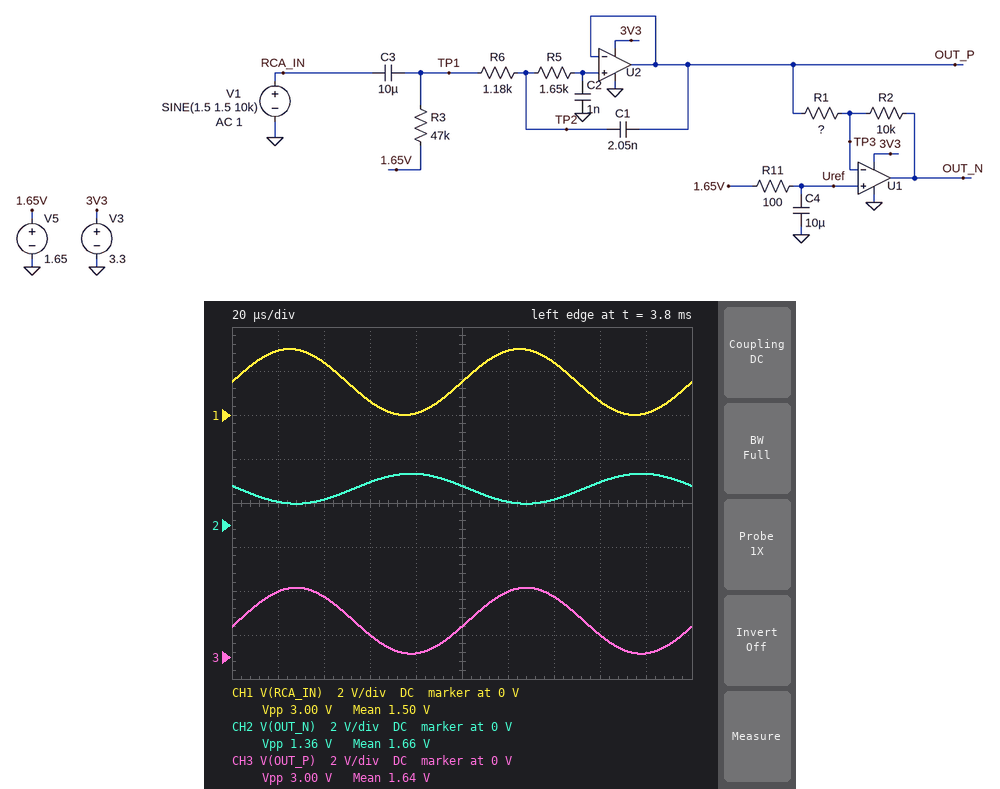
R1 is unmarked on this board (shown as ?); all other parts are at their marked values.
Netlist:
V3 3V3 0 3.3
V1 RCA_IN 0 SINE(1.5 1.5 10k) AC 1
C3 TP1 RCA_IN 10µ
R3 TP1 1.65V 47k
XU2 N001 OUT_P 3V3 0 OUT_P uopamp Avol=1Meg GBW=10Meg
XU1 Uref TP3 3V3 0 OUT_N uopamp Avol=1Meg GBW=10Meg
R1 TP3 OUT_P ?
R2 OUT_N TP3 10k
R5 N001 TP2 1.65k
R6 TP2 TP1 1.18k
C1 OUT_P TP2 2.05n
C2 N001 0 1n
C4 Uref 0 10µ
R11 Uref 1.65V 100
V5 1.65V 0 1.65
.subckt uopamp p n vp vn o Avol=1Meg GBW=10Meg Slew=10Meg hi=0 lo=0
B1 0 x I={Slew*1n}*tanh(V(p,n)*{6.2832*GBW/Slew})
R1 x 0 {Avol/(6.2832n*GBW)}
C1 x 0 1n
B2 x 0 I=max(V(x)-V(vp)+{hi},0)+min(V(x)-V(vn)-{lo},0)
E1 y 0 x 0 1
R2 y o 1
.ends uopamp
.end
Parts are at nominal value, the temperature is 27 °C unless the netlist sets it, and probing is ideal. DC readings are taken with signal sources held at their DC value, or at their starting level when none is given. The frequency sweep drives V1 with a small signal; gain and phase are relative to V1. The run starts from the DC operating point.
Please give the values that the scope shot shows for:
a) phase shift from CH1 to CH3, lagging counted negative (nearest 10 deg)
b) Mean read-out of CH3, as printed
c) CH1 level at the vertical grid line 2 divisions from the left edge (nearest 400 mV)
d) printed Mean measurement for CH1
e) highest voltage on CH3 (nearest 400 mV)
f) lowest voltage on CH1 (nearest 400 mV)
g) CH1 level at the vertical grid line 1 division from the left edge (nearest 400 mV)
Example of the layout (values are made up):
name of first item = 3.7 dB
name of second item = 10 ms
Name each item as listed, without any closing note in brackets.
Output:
phase shift from CH1 to CH3, lagging counted negative = -10 deg
Mean read-out of CH3, as printed = 1.64 V
CH1 level at the vertical grid line 2 divisions from the left edge = 2.4 V
printed Mean measurement for CH1 = 1.50 V
highest voltage on CH3 = 3.2 V
lowest voltage on CH1 = 0 V
CH1 level at the vertical grid line 1 division from the left edge = 2.8 V
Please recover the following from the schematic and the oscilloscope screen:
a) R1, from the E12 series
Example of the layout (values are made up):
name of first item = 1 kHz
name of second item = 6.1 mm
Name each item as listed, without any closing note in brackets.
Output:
R1, from the E12 series = 22 kΩ
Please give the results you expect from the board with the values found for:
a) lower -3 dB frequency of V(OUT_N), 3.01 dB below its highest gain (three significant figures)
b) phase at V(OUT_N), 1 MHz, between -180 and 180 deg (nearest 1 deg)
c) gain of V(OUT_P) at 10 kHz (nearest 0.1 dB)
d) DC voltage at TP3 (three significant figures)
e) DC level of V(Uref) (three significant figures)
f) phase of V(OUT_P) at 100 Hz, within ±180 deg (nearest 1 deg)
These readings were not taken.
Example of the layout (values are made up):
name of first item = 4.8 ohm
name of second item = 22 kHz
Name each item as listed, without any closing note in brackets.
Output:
lower -3 dB frequency of V(OUT_N), 3.01 dB below its highest gain = 339 mHz
phase at V(OUT_N), 1 MHz, between -180 and 180 deg = -8 deg
gain of V(OUT_P) at 10 kHz = 0 dB
DC voltage at TP3 = 1.65 V
DC level of V(Uref) = 1.65 V
phase of V(OUT_P) at 100 Hz, within ±180 deg = 0 deg
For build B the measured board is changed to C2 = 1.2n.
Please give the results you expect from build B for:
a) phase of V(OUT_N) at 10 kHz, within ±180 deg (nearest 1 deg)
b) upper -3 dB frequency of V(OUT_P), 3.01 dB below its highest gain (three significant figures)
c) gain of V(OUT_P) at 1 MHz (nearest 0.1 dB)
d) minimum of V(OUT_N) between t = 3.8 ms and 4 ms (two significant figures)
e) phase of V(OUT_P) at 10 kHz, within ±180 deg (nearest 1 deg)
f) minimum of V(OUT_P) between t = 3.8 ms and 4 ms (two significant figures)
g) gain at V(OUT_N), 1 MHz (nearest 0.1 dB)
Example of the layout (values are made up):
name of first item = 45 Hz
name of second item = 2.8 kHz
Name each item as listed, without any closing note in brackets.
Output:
phase of V(OUT_N) at 10 kHz, within ±180 deg = 168 deg
upper -3 dB frequency of V(OUT_P), 3.01 dB below its highest gain = 65.8 kHz
gain of V(OUT_P) at 1 MHz = -45.7 dB
minimum of V(OUT_N) between t = 3.8 ms and 4 ms = 970 mV
phase of V(OUT_P) at 10 kHz, within ±180 deg = -12 deg
minimum of V(OUT_P) between t = 3.8 ms and 4 ms = 160 mV
gain at V(OUT_N), 1 MHz = -52.6 dB
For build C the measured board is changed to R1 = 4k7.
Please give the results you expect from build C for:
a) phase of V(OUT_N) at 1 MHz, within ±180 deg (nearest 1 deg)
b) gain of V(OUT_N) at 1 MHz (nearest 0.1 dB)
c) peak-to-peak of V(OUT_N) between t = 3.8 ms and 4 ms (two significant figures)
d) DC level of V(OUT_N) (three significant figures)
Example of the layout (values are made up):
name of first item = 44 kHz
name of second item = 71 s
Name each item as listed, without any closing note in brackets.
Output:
phase of V(OUT_N) at 1 MHz, within ±180 deg = -17 deg
gain of V(OUT_N) at 1 MHz = -37.9 dB
peak-to-peak of V(OUT_N) between t = 3.8 ms and 4 ms = 3.3 V
DC level of V(OUT_N) = 1.65 V
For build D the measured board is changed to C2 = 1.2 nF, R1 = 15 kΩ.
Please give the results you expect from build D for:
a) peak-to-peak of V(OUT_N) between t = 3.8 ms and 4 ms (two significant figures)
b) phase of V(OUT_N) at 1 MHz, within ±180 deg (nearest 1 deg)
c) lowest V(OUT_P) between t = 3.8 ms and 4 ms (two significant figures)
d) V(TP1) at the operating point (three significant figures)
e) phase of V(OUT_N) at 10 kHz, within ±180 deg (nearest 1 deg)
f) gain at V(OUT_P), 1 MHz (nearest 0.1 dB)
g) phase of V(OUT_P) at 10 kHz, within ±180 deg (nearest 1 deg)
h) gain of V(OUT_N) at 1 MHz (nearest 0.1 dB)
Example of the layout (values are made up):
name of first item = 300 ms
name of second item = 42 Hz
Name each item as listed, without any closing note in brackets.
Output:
peak-to-peak of V(OUT_N) between t = 3.8 ms and 4 ms = 2.0 V
phase of V(OUT_N) at 1 MHz, within ±180 deg = -10 deg
lowest V(OUT_P) between t = 3.8 ms and 4 ms = 160 mV
V(TP1) at the operating point = 1.65 V
phase of V(OUT_N) at 10 kHz, within ±180 deg = 168 deg
gain at V(OUT_P), 1 MHz = -45.7 dB
phase of V(OUT_P) at 10 kHz, within ±180 deg = -12 deg
gain of V(OUT_N) at 1 MHz = -49.3 dB
